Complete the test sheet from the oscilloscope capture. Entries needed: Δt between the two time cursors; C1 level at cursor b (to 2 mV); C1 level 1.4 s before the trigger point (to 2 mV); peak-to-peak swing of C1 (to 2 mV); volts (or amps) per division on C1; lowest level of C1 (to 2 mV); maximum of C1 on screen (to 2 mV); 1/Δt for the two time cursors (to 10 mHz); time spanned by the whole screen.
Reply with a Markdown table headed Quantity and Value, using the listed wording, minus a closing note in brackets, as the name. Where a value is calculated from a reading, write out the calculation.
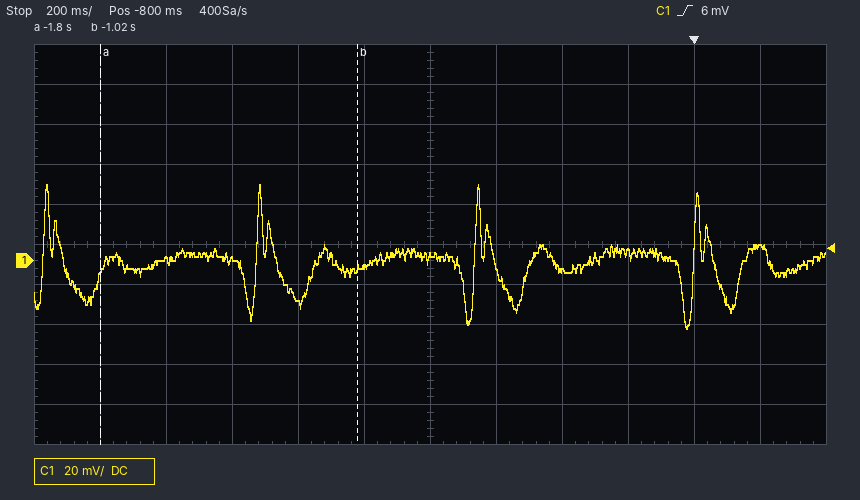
| Quantity | Value |
|---|---|
| Δt between the two time cursors | -1.02 s − (-1.8 s) = 780 ms |
| C1 level at cursor b | -4 mV |
| C1 level 1.4 s before the trigger point | 0 mV |
| peak-to-peak swing of C1 | 38 mV − (-34 mV) = 72 mV |
| volts (or amps) per division on C1 | 20 mV |
| lowest level of C1 | -34 mV |
| maximum of C1 on screen | 38 mV |
| 1/Δt for the two time cursors | 1 / 780 ms ≈ 1.28 Hz |
| time spanned by the whole screen | 2.4 s |
